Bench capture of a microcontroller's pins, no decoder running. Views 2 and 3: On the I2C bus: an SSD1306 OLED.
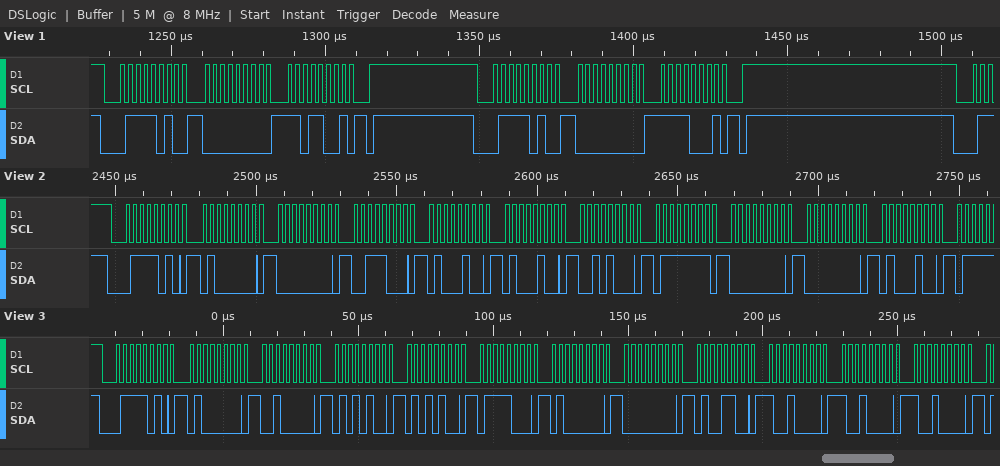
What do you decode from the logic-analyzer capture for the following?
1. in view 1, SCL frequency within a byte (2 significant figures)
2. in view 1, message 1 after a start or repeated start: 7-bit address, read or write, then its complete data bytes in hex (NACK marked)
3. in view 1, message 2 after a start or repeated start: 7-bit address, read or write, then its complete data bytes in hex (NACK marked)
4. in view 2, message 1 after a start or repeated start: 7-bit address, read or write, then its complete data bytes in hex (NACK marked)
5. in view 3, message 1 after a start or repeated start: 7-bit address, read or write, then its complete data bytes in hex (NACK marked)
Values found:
400 kHz
0x3D write: 00 D9
0x3D write: 00 F1
0x3D write: 40 00 38 44 44 28 7F 00 00 44
0x3D write: 40 20 54 54 78 40 00 4C 90 90 90
